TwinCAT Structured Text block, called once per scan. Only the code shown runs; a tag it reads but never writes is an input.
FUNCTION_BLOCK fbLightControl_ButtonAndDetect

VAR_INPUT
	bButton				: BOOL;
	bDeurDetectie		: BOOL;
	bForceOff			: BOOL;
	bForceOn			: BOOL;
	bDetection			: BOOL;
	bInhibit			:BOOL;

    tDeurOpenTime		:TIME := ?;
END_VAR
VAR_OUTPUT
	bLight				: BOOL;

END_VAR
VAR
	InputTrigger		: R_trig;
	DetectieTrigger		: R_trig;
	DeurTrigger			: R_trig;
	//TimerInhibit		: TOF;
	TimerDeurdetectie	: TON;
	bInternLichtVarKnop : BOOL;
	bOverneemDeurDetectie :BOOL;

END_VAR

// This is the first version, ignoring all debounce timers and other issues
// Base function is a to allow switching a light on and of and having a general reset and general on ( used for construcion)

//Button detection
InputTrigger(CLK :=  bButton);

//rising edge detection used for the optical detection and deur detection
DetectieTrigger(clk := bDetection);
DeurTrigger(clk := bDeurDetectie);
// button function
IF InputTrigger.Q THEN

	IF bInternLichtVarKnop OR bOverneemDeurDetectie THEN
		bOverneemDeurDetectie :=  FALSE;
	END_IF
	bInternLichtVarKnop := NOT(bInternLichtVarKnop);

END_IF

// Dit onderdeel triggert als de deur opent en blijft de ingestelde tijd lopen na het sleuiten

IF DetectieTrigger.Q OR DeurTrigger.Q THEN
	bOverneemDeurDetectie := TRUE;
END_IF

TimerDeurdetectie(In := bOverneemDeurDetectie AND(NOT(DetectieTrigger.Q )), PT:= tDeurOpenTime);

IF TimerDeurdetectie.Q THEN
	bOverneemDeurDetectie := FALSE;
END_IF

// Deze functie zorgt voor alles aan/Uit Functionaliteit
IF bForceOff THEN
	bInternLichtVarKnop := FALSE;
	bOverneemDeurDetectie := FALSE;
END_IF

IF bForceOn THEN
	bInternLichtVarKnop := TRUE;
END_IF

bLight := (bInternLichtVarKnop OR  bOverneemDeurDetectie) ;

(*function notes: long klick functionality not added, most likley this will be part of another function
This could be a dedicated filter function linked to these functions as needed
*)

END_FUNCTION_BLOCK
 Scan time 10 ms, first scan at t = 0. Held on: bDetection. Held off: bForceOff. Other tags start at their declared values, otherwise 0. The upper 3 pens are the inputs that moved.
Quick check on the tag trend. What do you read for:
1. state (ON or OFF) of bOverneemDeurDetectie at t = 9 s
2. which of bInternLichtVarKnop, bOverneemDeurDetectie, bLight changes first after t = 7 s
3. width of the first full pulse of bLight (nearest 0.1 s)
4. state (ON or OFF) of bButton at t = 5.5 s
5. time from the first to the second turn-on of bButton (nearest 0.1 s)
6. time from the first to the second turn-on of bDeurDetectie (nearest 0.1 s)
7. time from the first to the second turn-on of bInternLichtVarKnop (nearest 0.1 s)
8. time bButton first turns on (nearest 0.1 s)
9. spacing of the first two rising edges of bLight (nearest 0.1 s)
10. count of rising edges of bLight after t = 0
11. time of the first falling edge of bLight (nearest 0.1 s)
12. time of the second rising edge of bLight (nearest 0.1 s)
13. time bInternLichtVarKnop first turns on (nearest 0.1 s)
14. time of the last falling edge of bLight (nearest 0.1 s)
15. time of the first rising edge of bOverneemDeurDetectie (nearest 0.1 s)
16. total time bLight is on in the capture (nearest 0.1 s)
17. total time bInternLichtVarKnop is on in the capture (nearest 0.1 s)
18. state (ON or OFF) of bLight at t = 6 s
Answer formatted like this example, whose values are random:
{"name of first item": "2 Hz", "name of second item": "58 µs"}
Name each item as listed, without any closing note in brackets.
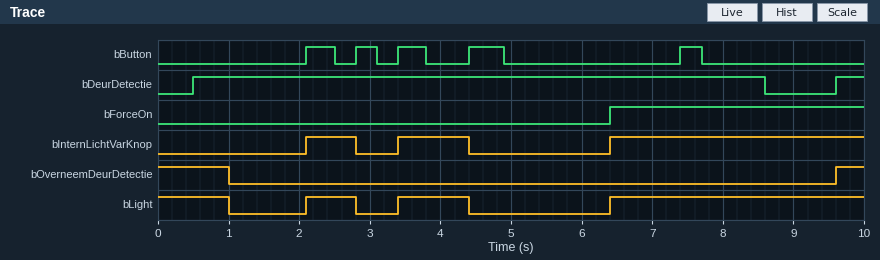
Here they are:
{"state (ON or OFF) of bOverneemDeurDetectie at t = 9 s": "OFF", "which of bInternLichtVarKnop, bOverneemDeurDetectie, bLight changes first after t = 7 s": "bOverneemDeurDetectie", "width of the first full pulse of bLight": "0.7 s", "state (ON or OFF) of bButton at t = 5.5 s": "OFF", "time from the first to the second turn-on of bButton": "0.7 s", "time from the first to the second turn-on of bDeurDetectie": "9.1 s", "time from the first to the second turn-on of bInternLichtVarKnop": "1.3 s", "time bButton first turns on": "2.1 s", "spacing of the first two rising edges of bLight": "1.3 s", "count of rising edges of bLight after t = 0": "3", "time of the first falling edge of bLight": "1.0 s", "time of the second rising edge of bLight": "3.4 s", "time bInternLichtVarKnop first turns on": "2.1 s", "time of the last falling edge of bLight": "4.4 s", "time of the first rising edge of bOverneemDeurDetectie": "9.6 s", "total time bLight is on in the capture": "6.3 s", "total time bInternLichtVarKnop is on in the capture": "5.3 s", "state (ON or OFF) of bLight at t = 6 s": "OFF"}
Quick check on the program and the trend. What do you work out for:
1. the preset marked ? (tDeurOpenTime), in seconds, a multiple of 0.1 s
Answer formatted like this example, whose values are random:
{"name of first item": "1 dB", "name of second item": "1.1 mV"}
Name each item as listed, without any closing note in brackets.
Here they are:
{"the preset marked ? (tDeurOpenTime), in seconds, a multiple of 0.1 s": "1.0 s"}
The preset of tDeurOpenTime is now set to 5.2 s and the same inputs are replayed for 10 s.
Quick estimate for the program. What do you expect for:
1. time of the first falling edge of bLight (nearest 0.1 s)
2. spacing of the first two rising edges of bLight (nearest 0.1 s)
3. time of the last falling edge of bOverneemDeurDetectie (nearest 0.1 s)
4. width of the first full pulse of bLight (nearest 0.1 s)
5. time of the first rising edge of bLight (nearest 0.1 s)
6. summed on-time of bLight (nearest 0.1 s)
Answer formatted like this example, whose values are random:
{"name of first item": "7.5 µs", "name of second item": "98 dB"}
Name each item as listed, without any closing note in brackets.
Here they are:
{"time of the first falling edge of bLight": "2.8 s", "spacing of the first two rising edges of bLight": "3.0 s", "time of the last falling edge of bOverneemDeurDetectie": "2.1 s", "width of the first full pulse of bLight": "1.0 s", "time of the first rising edge of bLight": "3.4 s", "summed on-time of bLight": "7.4 s"}
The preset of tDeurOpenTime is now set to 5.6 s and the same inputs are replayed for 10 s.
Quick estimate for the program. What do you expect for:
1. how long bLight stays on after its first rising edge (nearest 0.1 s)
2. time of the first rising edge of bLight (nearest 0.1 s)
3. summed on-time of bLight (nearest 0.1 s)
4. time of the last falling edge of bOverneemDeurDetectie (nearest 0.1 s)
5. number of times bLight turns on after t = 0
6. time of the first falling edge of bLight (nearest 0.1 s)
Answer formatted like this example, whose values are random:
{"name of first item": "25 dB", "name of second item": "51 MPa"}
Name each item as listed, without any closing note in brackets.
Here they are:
{"how long bLight stays on after its first rising edge": "1.0 s", "time of the first rising edge of bLight": "3.4 s", "summed on-time of bLight": "7.4 s", "time of the last falling edge of bOverneemDeurDetectie": "2.1 s", "number of times bLight turns on after t = 0": "2", "time of the first falling edge of bLight": "2.8 s"}
